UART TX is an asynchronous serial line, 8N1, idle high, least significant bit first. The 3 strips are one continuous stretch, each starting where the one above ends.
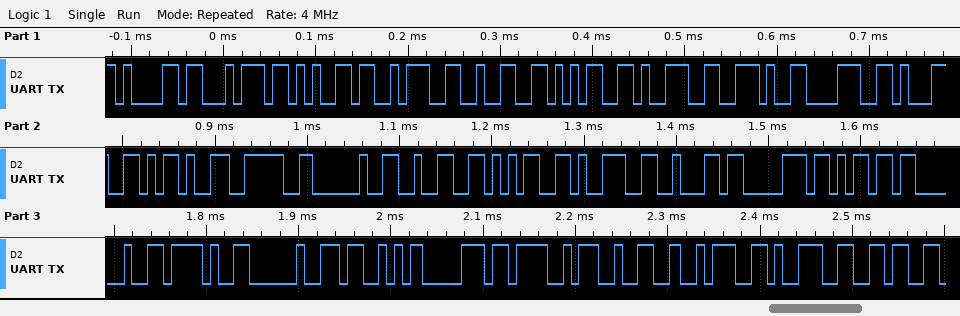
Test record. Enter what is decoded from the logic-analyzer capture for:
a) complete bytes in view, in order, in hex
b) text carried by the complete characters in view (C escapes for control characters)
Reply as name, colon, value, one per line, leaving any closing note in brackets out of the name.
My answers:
complete bytes in view, in order, in hex: 61 74 65 3A 32 35 39 2E 38 31 2D 3E 20 32 35 39 62 70 6D 20 2F 20 53 70 4F 32 3A 39 36
text carried by the complete characters in view: "ate:259.81-> 259bpm / SpO2:96"
